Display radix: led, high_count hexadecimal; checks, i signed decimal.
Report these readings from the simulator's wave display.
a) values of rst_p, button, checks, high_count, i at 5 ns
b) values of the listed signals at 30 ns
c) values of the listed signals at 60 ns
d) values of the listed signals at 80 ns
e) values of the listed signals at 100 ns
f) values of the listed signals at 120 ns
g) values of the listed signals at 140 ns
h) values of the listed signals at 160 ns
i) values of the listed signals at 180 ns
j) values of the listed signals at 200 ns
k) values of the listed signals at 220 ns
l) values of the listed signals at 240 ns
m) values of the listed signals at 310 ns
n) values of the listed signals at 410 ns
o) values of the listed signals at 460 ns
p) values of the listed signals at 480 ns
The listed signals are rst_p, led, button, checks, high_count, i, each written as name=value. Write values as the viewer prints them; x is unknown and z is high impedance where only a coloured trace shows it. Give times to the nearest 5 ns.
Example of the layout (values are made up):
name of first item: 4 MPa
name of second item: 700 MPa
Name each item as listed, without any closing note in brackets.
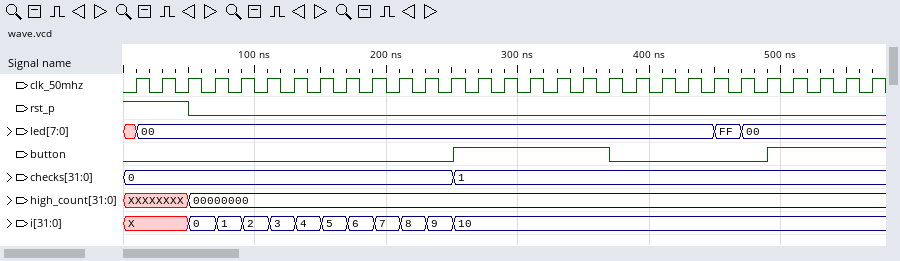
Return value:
values of rst_p, button, checks, high_count, i at 5 ns: rst_p=1, button=0, checks=0, high_count=XXXXXXXX, i=X
values of the listed signals at 30 ns: rst_p=1, led=00, button=0, checks=0, high_count=XXXXXXXX, i=X
values of the listed signals at 60 ns: rst_p=0, led=00, button=0, checks=0, high_count=00000000, i=0
values of the listed signals at 80 ns: rst_p=0, led=00, button=0, checks=0, high_count=00000000, i=1
values of the listed signals at 100 ns: rst_p=0, led=00, button=0, checks=0, high_count=00000000, i=2
values of the listed signals at 120 ns: rst_p=0, led=00, button=0, checks=0, high_count=00000000, i=3
values of the listed signals at 140 ns: rst_p=0, led=00, button=0, checks=0, high_count=00000000, i=4
values of the listed signals at 160 ns: rst_p=0, led=00, button=0, checks=0, high_count=00000000, i=5
values of the listed signals at 180 ns: rst_p=0, led=00, button=0, checks=0, high_count=00000000, i=6
values of the listed signals at 200 ns: rst_p=0, led=00, button=0, checks=0, high_count=00000000, i=7
values of the listed signals at 220 ns: rst_p=0, led=00, button=0, checks=0, high_count=00000000, i=8
values of the listed signals at 240 ns: rst_p=0, led=00, button=0, checks=0, high_count=00000000, i=9
values of the listed signals at 310 ns: rst_p=0, led=00, button=1, checks=1, high_count=00000000, i=10
values of the listed signals at 410 ns: rst_p=0, led=00, button=0, checks=1, high_count=00000000, i=10
values of the listed signals at 460 ns: rst_p=0, led=FF, button=0, checks=1, high_count=00000000, i=10
values of the listed signals at 480 ns: rst_p=0, led=00, button=0, checks=1, high_count=00000000, i=10
